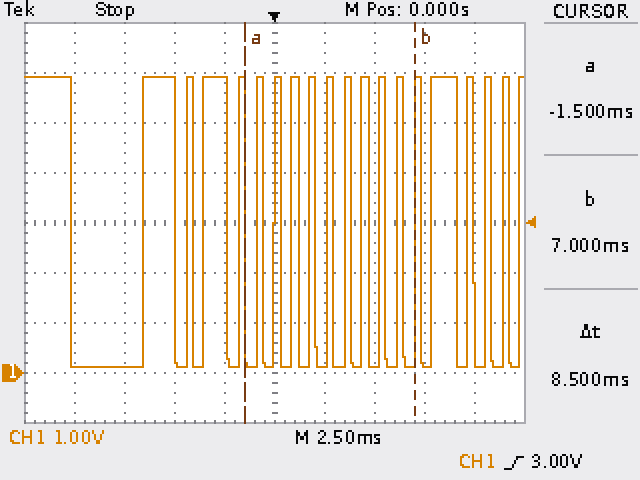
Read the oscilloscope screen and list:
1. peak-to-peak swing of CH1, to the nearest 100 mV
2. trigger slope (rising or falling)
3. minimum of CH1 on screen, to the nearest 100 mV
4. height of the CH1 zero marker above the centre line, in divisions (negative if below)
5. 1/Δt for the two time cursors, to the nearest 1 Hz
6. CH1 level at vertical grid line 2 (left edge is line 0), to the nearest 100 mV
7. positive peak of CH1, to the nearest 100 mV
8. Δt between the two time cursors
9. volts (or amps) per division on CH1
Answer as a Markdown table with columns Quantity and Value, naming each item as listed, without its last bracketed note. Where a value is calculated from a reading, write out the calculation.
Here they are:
| Quantity | Value |
|---|---|
| peak-to-peak swing of CH1, to the nearest 100 mV | 5.9 V − (100 mV) = 5.8 V |
| trigger slope | rising |
| minimum of CH1 on screen, to the nearest 100 mV | 100 mV |
| height of the CH1 zero marker above the centre line, in divisions | -3.0 div |
| 1/Δt for the two time cursors, to the nearest 1 Hz | 1 / 8.5 ms ≈ 118 Hz |
| CH1 level at vertical grid line 2 (left edge is line 0), to the nearest 100 mV | 100 mV |
| positive peak of CH1, to the nearest 100 mV | 5.9 V |
| Δt between the two time cursors | 8.5 ms |
| volts (or amps) per division on CH1 | 1 V |
